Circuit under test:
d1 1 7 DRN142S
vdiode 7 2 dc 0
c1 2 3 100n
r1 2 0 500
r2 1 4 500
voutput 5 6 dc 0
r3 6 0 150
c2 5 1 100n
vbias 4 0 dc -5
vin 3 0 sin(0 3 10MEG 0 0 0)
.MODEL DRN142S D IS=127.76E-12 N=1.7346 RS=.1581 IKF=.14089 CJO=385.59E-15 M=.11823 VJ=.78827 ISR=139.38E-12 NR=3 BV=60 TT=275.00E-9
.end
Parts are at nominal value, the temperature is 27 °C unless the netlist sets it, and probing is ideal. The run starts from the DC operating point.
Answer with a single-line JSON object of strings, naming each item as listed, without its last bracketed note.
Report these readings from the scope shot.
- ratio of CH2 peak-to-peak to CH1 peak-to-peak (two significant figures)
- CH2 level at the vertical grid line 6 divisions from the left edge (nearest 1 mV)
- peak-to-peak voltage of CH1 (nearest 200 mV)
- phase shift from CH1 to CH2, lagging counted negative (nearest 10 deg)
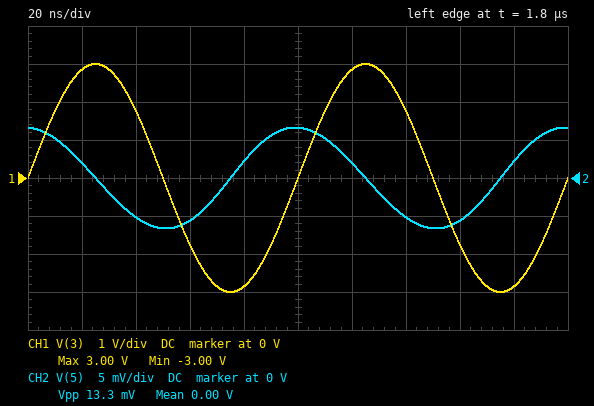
{"ratio of CH2 peak-to-peak to CH1 peak-to-peak": "0.0022", "CH2 level at the vertical grid line 6 divisions from the left edge": "2 mV", "peak-to-peak voltage of CH1": "6.0 V", "phase shift from CH1 to CH2, lagging counted negative": "90 deg"}
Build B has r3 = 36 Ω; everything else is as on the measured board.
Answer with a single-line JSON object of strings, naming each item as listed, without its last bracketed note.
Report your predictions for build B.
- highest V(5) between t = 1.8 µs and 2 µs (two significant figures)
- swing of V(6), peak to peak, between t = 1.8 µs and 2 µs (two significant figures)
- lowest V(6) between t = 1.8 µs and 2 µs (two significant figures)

{"highest V(5) between t = 1.8 µs and 2 µs": "1.9 mV", "swing of V(6), peak to peak, between t = 1.8 µs and 2 µs": "3.9 mV", "lowest V(6) between t = 1.8 µs and 2 µs": "-1.9 mV"}
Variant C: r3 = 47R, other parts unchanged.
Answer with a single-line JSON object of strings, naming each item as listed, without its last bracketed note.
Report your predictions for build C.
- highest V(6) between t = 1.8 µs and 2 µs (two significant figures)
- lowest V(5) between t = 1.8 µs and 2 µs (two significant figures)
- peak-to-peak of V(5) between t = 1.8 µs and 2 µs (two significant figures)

{"highest V(6) between t = 1.8 µs and 2 µs": "2.5 mV", "lowest V(5) between t = 1.8 µs and 2 µs": "-2.5 mV", "peak-to-peak of V(5) between t = 1.8 µs and 2 µs": "4.9 mV"}
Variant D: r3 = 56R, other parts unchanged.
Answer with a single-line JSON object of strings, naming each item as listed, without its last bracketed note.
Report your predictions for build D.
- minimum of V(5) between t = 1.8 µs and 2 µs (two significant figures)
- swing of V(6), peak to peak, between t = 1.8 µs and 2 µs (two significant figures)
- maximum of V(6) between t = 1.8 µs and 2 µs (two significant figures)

{"minimum of V(5) between t = 1.8 µs and 2 µs": "-2.9 mV", "swing of V(6), peak to peak, between t = 1.8 µs and 2 µs": "5.8 mV", "maximum of V(6) between t = 1.8 µs and 2 µs": "2.9 mV"}
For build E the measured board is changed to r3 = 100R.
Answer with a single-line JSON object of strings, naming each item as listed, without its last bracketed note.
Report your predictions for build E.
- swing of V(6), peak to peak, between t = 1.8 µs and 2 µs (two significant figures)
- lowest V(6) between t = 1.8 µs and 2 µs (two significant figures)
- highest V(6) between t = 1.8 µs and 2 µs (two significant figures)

{"swing of V(6), peak to peak, between t = 1.8 µs and 2 µs": "9.6 mV", "lowest V(6) between t = 1.8 µs and 2 µs": "-4.8 mV", "highest V(6) between t = 1.8 µs and 2 µs": "4.8 mV"}
